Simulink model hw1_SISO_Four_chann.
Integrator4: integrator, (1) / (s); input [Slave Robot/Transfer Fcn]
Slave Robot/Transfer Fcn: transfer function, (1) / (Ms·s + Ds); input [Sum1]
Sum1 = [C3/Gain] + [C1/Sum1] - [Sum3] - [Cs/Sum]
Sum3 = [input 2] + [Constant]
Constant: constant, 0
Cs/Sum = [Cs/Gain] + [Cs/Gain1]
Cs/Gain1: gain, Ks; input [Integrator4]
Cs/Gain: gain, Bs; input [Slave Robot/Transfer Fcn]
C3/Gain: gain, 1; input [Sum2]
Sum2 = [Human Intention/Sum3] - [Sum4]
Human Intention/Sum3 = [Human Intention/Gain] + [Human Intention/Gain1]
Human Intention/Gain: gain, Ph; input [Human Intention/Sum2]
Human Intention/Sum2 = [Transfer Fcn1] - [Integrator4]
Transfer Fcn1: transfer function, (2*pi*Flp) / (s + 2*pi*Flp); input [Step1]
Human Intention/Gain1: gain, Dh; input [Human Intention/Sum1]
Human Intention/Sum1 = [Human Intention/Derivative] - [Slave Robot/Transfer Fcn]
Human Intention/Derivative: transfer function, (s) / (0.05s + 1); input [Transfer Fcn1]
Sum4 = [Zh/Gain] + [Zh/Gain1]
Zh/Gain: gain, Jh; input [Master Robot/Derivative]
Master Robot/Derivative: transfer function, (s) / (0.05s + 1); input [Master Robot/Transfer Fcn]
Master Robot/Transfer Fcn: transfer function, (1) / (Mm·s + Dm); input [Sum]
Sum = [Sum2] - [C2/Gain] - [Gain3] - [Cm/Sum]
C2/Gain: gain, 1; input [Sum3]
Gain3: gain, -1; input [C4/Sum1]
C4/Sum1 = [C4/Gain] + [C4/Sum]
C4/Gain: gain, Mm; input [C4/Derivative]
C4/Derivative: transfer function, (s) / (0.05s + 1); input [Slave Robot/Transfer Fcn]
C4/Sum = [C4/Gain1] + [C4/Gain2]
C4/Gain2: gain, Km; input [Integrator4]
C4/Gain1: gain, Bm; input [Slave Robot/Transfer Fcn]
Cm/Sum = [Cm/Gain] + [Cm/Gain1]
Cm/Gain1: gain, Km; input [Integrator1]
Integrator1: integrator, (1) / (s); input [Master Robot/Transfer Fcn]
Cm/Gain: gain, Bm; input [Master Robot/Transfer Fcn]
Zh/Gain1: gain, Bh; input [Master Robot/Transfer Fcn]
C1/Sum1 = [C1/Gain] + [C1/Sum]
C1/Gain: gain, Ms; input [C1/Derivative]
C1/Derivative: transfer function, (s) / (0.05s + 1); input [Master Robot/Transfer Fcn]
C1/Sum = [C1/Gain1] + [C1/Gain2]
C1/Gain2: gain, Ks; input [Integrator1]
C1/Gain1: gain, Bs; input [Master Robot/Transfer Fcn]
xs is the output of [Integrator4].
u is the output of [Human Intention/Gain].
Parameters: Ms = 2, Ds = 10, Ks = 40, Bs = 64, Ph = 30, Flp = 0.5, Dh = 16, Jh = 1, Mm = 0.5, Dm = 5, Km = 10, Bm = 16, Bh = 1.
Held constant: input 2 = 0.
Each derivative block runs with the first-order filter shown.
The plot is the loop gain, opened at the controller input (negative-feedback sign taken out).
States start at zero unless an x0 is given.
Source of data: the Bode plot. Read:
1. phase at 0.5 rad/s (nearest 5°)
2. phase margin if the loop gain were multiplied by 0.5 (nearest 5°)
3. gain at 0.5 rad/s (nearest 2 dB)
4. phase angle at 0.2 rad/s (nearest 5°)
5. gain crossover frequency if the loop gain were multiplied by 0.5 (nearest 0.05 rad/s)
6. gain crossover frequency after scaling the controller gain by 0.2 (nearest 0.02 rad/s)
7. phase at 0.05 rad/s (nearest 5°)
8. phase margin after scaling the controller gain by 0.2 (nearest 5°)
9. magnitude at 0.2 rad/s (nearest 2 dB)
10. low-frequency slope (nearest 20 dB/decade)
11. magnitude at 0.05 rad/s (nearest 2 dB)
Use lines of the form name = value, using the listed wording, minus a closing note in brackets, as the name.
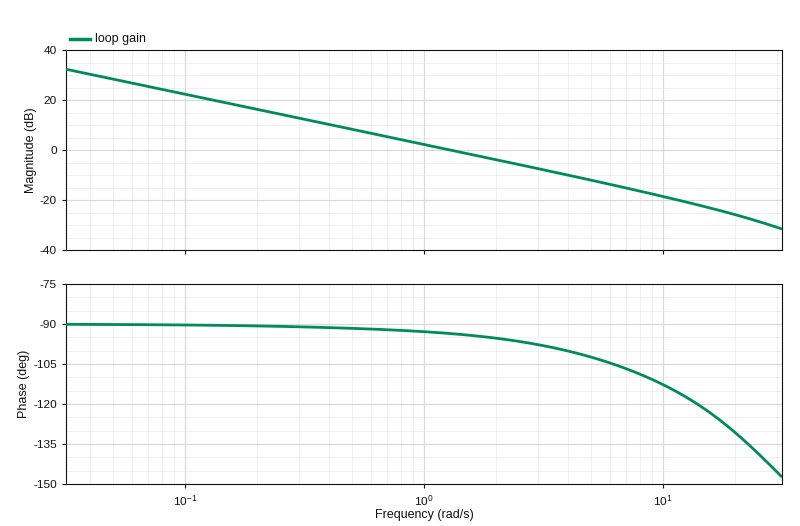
phase at 0.5 rad/s = -90°
phase margin if the loop gain were multiplied by 0.5 = 90°
gain at 0.5 rad/s = 8 dB
phase angle at 0.2 rad/s = -90°
gain crossover frequency if the loop gain were multiplied by 0.5 = 0.65 rad/s
gain crossover frequency after scaling the controller gain by 0.2 = 0.26 rad/s
phase at 0.05 rad/s = -90°
phase margin after scaling the controller gain by 0.2 = 90°
magnitude at 0.2 rad/s = 16 dB
low-frequency slope = -20 dB/decade
magnitude at 0.05 rad/s = 28 dB
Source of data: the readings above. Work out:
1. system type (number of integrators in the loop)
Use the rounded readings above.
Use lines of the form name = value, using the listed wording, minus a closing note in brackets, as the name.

system type = 1
